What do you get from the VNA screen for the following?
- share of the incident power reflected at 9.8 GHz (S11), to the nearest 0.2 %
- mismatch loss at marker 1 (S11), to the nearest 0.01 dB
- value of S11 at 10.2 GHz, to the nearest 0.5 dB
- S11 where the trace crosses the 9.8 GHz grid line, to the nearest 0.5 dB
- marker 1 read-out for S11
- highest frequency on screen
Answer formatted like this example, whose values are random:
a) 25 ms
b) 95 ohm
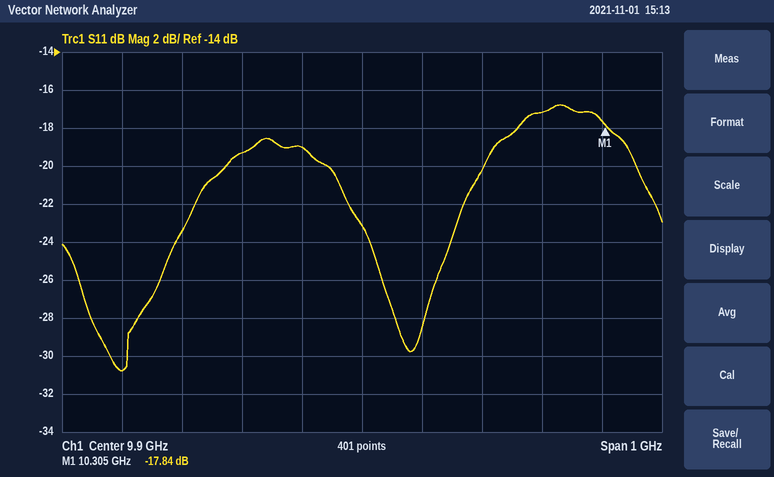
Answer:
a) 1.2 %
b) 0.07 dB
c) -17.0 dB
d) -19.0 dB
e) -17.84 dB
f) 10.4 GHz
